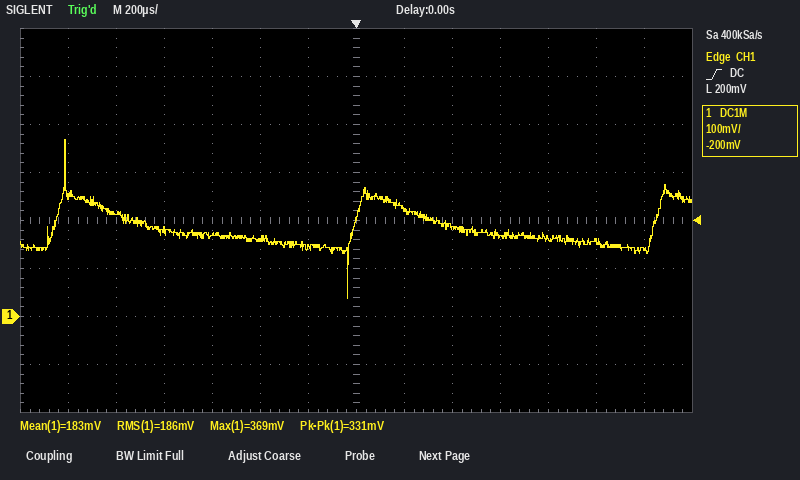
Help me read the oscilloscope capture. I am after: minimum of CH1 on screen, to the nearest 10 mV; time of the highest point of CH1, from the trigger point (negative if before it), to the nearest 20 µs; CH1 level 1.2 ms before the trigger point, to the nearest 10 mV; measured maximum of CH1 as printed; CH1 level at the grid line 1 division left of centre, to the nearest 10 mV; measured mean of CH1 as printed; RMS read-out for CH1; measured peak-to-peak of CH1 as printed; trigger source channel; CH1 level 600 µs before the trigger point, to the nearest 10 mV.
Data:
40 mV
-1.22 ms
250 mV
369 mV
140 mV
183 mV
186 mV
331 mV
CH1
170 mV
